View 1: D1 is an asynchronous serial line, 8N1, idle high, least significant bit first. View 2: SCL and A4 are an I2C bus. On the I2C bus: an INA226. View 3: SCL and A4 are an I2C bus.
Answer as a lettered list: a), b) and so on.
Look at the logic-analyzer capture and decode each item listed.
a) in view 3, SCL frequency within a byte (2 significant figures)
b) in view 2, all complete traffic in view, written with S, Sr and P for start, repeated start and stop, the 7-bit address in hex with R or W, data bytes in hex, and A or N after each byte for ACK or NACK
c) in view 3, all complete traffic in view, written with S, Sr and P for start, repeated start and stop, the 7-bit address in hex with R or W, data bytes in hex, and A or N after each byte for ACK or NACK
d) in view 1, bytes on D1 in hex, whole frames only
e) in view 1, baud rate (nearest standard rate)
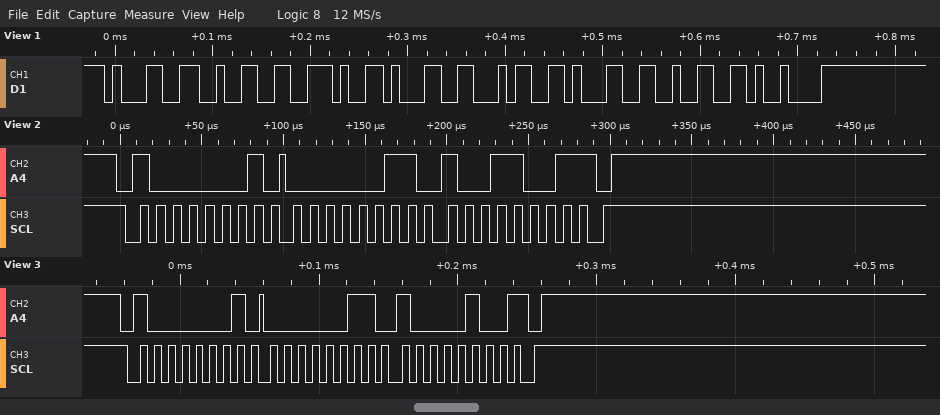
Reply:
a) 100 kHz
b) S 40R A 03 A 99 N P
c) S 40R A 03 A 84 N P
d) 31 32 2E 31 34 31 32 09
e) 115200 baud
